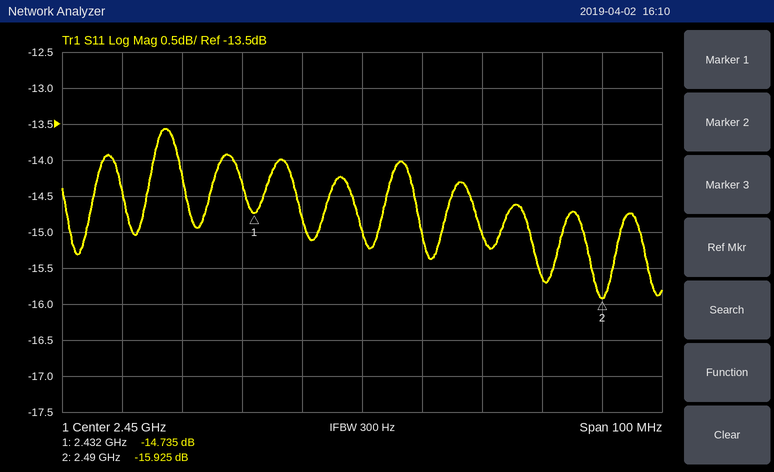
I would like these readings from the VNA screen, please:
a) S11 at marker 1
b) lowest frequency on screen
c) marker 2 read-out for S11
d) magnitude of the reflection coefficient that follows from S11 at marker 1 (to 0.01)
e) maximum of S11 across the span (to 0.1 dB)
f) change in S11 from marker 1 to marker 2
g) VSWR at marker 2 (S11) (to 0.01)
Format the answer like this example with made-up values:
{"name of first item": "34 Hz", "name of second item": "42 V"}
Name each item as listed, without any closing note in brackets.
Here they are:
{"S11 at marker 1": "-14.735 dB", "lowest frequency on screen": "2.4 GHz", "marker 2 read-out for S11": "-15.925 dB", "magnitude of the reflection coefficient that follows from S11 at marker 1": "0.18", "maximum of S11 across the span": "-13.6 dB", "change in S11 from marker 1 to marker 2": "-1.190 dB", "VSWR at marker 2 (S11)": "1.38"}
